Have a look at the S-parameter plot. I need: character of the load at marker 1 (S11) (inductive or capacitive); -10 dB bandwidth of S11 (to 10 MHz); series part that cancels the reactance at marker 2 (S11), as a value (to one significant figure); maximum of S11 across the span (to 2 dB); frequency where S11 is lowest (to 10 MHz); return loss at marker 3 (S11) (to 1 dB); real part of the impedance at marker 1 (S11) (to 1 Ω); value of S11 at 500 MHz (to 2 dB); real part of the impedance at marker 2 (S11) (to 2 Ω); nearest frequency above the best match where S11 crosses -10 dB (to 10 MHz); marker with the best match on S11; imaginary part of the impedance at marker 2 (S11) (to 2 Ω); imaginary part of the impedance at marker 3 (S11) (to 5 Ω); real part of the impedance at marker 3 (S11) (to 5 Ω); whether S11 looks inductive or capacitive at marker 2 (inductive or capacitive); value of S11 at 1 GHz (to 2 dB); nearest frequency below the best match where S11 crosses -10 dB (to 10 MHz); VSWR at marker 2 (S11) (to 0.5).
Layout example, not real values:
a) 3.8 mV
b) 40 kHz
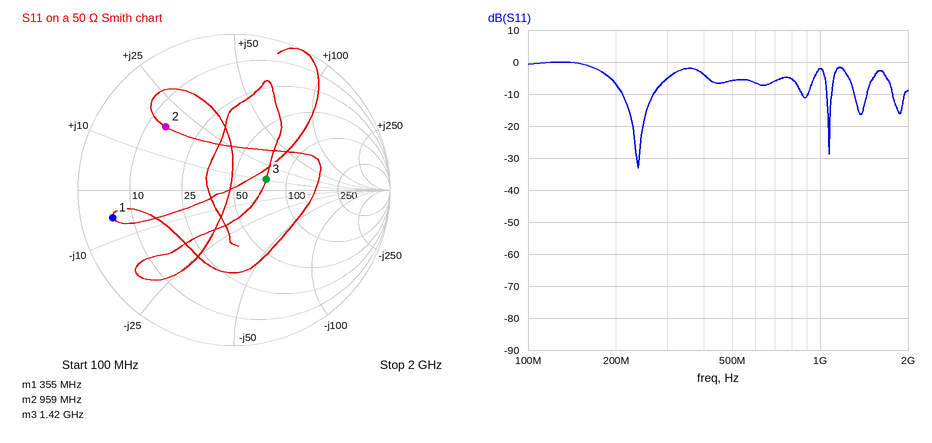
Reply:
a) capacitive
b) 60 MHz
c) 9 pF
d) 0 dB
e) 240 MHz
f) 13 dB
g) 6 Ω
h) -6 dB
i) 14 Ω
j) 270 MHz
k) marker 3
l) +18 Ω
m) +10 Ω
n) 75 Ω
o) inductive
p) -2 dB
q) 210 MHz
r) 4.0
